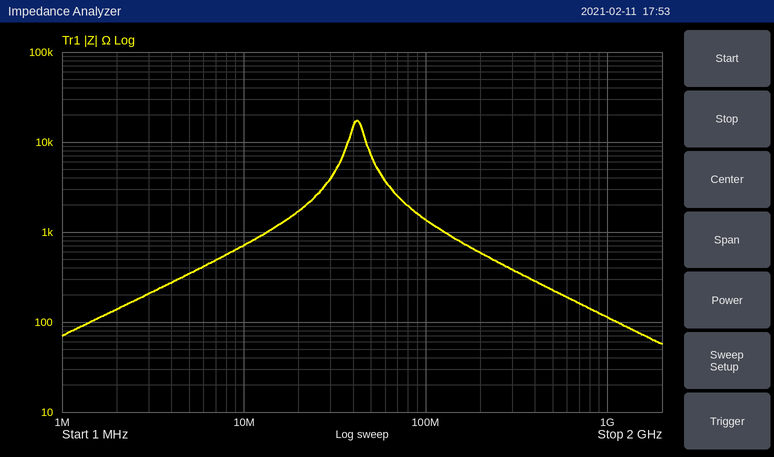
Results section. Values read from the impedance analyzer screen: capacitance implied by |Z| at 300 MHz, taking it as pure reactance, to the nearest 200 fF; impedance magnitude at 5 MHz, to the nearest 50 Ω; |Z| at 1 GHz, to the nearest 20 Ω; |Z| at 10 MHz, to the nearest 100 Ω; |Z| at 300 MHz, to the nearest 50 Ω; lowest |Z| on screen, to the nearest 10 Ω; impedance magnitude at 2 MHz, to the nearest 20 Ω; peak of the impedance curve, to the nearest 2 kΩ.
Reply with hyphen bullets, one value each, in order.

- 1.4 pF
- 350 Ω
- 120 Ω
- 700 Ω
- 400 Ω
- 60 Ω
- 140 Ω
- 18 kΩ
